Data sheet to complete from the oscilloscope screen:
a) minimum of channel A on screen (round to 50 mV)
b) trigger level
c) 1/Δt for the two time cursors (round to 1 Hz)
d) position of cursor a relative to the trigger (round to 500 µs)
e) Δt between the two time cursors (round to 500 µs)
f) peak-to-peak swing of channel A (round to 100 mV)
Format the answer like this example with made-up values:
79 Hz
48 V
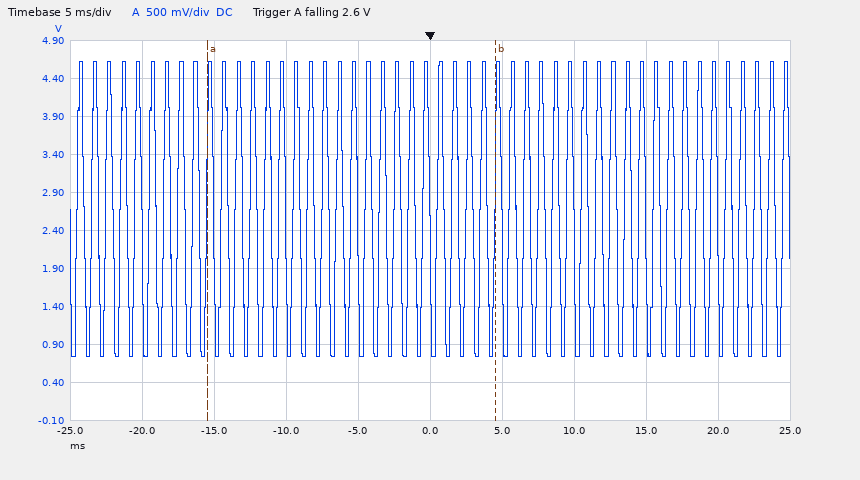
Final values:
750 mV
2.6 V
50 Hz
-15.5 ms
20.0 ms
3.90 V
